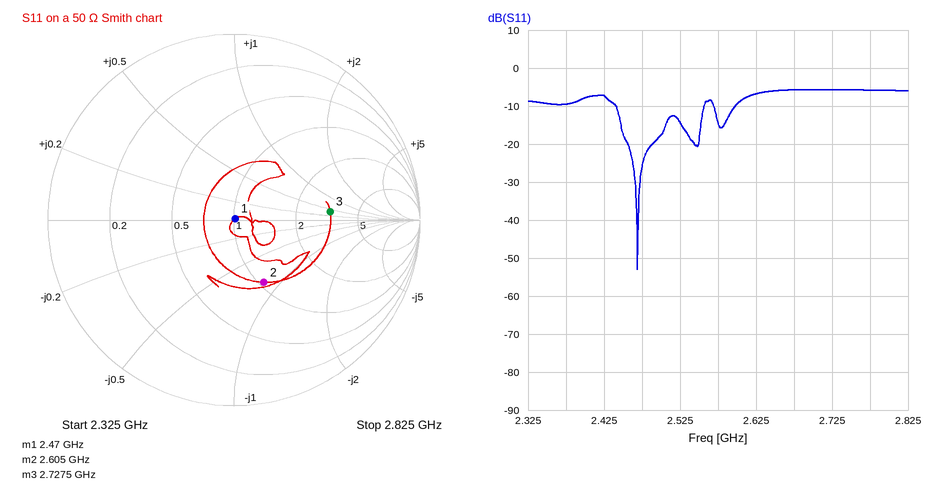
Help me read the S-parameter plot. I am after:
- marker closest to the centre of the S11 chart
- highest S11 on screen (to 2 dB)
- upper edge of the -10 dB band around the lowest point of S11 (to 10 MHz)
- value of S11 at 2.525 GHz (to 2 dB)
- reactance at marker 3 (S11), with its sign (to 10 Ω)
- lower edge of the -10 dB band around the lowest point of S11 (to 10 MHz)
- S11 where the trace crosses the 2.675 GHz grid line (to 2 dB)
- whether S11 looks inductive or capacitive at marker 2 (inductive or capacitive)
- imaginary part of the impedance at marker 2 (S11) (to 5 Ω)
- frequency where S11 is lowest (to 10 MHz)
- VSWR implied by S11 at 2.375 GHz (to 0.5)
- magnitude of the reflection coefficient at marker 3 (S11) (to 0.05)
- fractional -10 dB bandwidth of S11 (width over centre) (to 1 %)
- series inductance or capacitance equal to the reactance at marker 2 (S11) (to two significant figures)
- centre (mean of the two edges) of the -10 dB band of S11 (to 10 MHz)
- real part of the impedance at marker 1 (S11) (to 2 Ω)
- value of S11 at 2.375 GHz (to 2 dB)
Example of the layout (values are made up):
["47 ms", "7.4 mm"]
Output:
["marker 1", "-6 dB", "2.56 GHz", "-14 dB", "+20 Ω", "2.44 GHz", "-6 dB", "capacitive", "-40 Ω", "2.47 GHz", "2.0", "0.50", "5 %", "1.5 pF", "2.50 GHz", "50 Ω", "-10 dB"]
